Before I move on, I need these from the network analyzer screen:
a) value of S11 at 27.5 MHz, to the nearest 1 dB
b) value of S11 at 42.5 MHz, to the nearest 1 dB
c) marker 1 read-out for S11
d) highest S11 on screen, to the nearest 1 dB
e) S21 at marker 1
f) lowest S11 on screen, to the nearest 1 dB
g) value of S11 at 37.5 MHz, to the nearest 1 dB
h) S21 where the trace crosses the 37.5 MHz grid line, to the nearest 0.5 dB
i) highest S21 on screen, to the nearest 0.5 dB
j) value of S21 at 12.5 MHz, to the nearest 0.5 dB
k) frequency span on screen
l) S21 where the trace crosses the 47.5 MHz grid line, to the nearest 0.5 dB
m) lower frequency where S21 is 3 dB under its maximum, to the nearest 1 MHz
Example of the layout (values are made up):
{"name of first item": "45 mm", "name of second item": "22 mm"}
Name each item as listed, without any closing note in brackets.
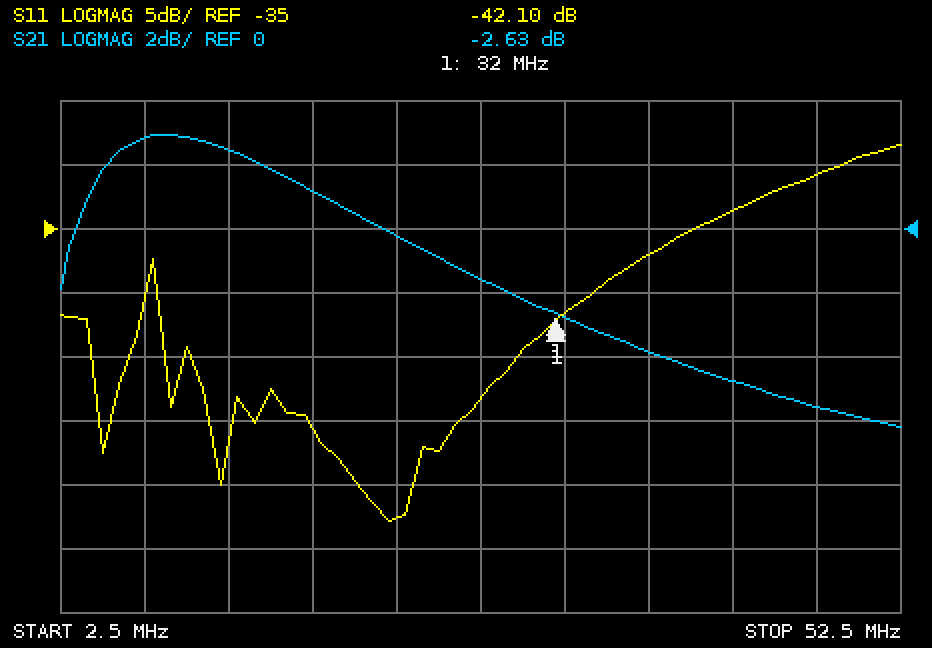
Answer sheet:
{"value of S11 at 27.5 MHz, to the nearest 1 dB": "-48 dB", "value of S11 at 42.5 MHz, to the nearest 1 dB": "-34 dB", "marker 1 read-out for S11": "-42.10 dB", "highest S11 on screen, to the nearest 1 dB": "-28 dB", "S21 at marker 1": "-2.63 dB", "lowest S11 on screen, to the nearest 1 dB": "-58 dB", "value of S11 at 37.5 MHz, to the nearest 1 dB": "-37 dB", "S21 where the trace crosses the 37.5 MHz grid line, to the nearest 0.5 dB": "-4.0 dB", "highest S21 on screen, to the nearest 0.5 dB": "3.0 dB", "value of S21 at 12.5 MHz, to the nearest 0.5 dB": "2.5 dB", "frequency span on screen": "50 MHz", "S21 where the trace crosses the 47.5 MHz grid line, to the nearest 0.5 dB": "-5.5 dB", "lower frequency where S21 is 3 dB under its maximum, to the nearest 1 MHz": "3 MHz"}
